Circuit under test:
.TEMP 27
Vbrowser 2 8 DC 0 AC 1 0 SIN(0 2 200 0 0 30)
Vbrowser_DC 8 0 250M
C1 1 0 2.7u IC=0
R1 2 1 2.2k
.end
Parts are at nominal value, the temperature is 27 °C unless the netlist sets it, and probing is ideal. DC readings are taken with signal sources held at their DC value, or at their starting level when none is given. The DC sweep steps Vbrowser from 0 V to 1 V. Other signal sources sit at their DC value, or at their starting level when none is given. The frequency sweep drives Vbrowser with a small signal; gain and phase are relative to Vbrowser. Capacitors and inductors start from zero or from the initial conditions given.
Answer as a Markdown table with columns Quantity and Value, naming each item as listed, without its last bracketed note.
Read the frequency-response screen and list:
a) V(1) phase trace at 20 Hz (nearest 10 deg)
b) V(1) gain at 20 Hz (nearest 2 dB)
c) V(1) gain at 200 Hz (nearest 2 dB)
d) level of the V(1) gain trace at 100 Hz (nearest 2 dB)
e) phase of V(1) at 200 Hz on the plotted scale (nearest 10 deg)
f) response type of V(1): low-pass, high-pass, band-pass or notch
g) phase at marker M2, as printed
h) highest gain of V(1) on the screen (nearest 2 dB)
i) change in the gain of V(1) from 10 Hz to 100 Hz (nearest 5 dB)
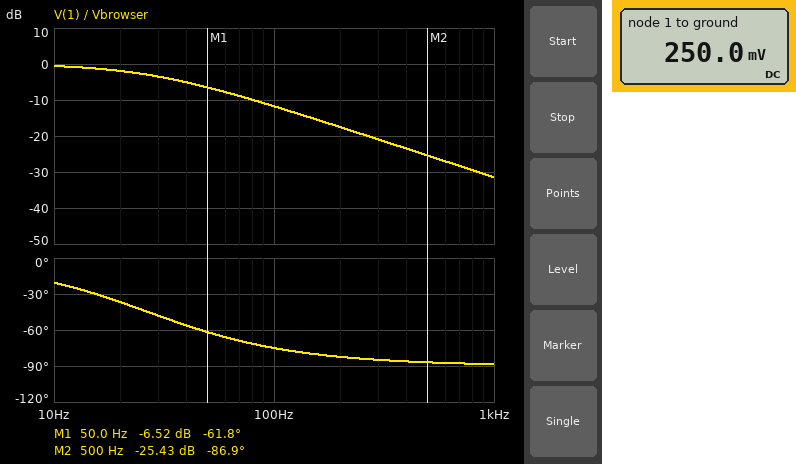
| Quantity | Value |
|---|---|
| V(1) phase trace at 20 Hz | -40 deg |
| V(1) gain at 20 Hz | -2 dB |
| V(1) gain at 200 Hz | -18 dB |
| level of the V(1) gain trace at 100 Hz | -12 dB |
| phase of V(1) at 200 Hz on the plotted scale | -80 deg |
| response type of V(1): low-pass, high-pass, band-pass or notch | low-pass |
| phase at marker M2, as printed | -86.9 deg |
| highest gain of V(1) on the screen | 0 dB |
| change in the gain of V(1) from 10 Hz to 100 Hz | -10 dB |
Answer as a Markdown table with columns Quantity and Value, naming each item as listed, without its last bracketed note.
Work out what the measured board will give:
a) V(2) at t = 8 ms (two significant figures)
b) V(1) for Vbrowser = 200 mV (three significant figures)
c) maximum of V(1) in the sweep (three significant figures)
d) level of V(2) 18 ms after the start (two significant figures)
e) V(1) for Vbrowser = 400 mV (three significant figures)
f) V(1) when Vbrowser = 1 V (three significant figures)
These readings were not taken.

| Quantity | Value |
|---|---|
| V(2) at t = 8 ms | -1.6 V |
| V(1) for Vbrowser = 200 mV | 450 mV |
| maximum of V(1) in the sweep | 1.25 V |
| level of V(2) 18 ms after the start | -1.6 V |
| V(1) for Vbrowser = 400 mV | 650 mV |
| V(1) when Vbrowser = 1 V | 1.25 V |
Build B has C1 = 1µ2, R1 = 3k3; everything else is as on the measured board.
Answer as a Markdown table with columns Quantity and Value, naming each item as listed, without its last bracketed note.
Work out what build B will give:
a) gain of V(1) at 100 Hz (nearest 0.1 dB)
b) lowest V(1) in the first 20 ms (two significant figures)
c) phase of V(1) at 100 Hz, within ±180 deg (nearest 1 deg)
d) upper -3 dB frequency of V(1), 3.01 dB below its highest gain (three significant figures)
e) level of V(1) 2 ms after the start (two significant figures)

| Quantity | Value |
|---|---|
| gain of V(1) at 100 Hz | -8.6 dB |
| lowest V(1) in the first 20 ms | -140 mV |
| phase of V(1) at 100 Hz, within ±180 deg | -68 deg |
| upper -3 dB frequency of V(1), 3.01 dB below its highest gain | 40.2 Hz |
| level of V(1) 2 ms after the start | 670 mV |
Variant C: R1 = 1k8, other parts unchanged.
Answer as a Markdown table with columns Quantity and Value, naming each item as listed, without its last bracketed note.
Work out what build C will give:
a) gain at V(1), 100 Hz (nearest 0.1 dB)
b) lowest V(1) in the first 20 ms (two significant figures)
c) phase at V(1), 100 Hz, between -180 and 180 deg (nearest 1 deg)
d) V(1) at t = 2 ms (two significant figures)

| Quantity | Value |
|---|---|
| gain at V(1), 100 Hz | -10.1 dB |
| lowest V(1) in the first 20 ms | -73 mV |
| phase at V(1), 100 Hz, between -180 and 180 deg | -72 deg |
| V(1) at t = 2 ms | 570 mV |
